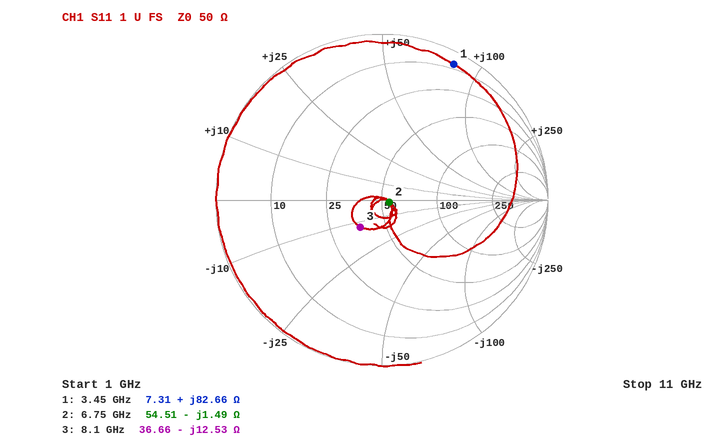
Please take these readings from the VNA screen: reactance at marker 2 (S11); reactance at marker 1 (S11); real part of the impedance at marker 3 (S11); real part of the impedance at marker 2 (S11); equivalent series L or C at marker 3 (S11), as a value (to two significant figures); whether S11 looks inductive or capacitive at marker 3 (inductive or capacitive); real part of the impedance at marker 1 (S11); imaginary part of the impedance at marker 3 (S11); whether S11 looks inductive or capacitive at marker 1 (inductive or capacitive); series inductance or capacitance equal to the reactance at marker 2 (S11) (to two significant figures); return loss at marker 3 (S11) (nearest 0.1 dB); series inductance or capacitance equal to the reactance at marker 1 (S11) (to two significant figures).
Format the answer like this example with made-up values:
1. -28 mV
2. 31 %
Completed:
1. -1.49 Ω
2. +82.66 Ω
3. 36.66 Ω
4. 54.51 Ω
5. 1.6 pF
6. capacitive
7. 7.31 Ω
8. -12.53 Ω
9. inductive
10. 16 pF
11. 13.6 dB
12. 3.8 nH
